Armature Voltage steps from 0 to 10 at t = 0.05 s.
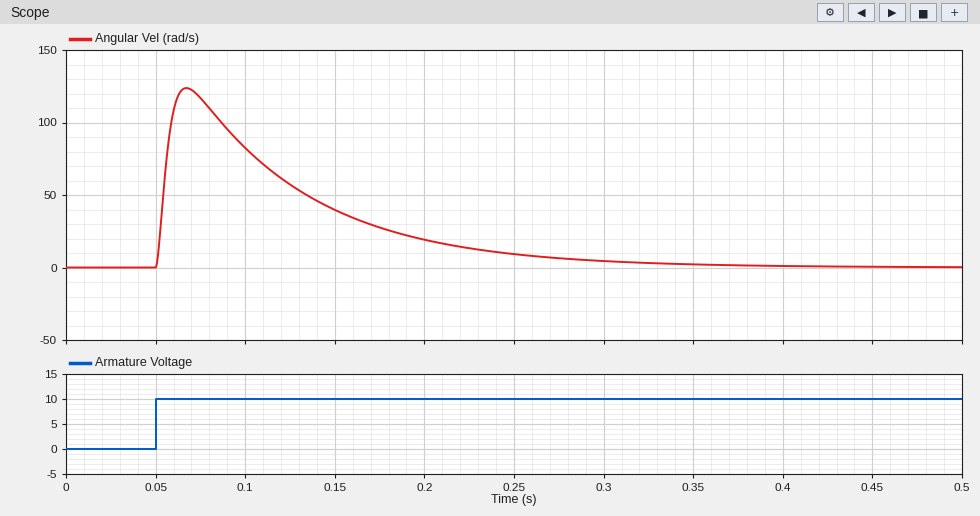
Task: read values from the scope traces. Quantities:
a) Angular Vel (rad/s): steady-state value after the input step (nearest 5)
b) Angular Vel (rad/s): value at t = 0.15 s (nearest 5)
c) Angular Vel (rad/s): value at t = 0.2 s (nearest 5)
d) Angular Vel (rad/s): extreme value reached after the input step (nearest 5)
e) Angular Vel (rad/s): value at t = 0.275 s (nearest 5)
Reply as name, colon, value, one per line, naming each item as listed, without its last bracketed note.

Angular Vel (rad/s): steady-state value after the input step: 0
Angular Vel (rad/s): value at t = 0.15 s: 40
Angular Vel (rad/s): value at t = 0.2 s: 20
Angular Vel (rad/s): extreme value reached after the input step: 125
Angular Vel (rad/s): value at t = 0.275 s: 5
